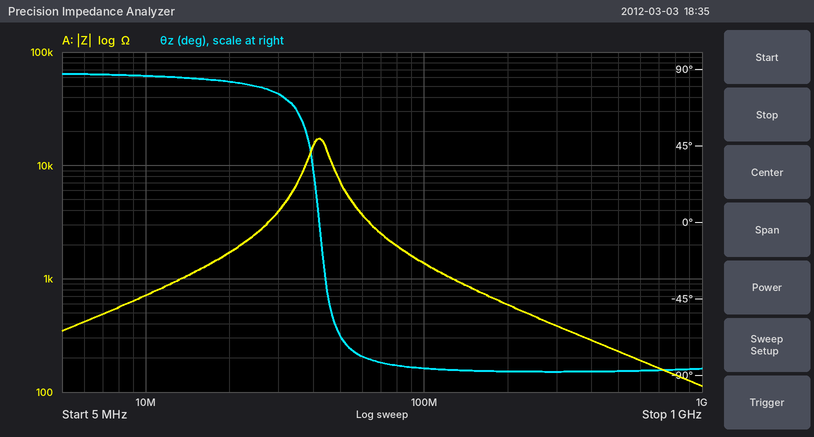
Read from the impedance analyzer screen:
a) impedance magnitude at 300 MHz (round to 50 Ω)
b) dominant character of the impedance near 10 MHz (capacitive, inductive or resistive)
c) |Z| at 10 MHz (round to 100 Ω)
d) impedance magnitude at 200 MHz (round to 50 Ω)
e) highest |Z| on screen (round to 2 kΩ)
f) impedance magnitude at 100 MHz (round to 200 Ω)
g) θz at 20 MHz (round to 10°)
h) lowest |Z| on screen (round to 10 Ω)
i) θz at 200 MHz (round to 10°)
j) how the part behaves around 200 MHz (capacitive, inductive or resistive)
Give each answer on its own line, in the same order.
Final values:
400 Ω
inductive
700 Ω
600 Ω
18 kΩ
1.4 kΩ
80°
110 Ω
-90°
capacitive
